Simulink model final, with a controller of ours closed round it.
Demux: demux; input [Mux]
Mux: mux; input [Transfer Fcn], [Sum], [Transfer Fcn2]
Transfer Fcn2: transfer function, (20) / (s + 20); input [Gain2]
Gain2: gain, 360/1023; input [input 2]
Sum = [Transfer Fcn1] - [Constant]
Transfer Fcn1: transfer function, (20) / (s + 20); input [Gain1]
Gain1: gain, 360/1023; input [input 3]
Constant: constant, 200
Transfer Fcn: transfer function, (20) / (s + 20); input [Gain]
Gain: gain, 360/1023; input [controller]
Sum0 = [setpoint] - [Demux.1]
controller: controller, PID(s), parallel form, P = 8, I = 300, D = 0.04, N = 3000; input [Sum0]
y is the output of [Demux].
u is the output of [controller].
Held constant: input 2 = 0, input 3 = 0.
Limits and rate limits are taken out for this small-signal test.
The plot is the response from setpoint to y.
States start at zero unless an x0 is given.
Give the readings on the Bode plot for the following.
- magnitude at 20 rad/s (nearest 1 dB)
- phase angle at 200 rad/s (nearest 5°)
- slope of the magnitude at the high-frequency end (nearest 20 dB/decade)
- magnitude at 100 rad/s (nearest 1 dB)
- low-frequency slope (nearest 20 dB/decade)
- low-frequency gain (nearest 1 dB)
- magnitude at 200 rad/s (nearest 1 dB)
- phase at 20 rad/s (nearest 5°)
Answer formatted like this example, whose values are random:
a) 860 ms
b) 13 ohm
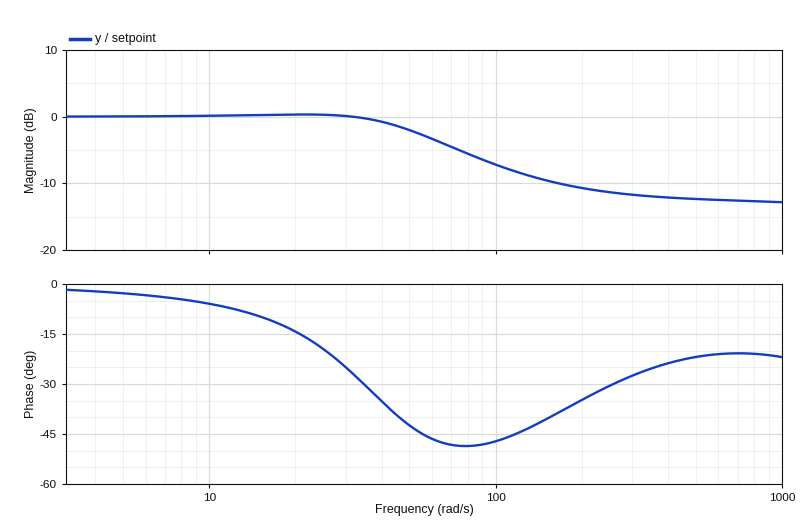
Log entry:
a) 0 dB
b) -35°
c) 0 dB/decade
d) -7 dB
e) 0 dB/decade
f) 0 dB
g) -11 dB
h) -15°
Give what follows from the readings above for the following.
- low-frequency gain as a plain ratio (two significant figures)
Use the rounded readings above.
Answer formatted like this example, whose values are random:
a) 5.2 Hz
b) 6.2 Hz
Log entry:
a) 1.0
